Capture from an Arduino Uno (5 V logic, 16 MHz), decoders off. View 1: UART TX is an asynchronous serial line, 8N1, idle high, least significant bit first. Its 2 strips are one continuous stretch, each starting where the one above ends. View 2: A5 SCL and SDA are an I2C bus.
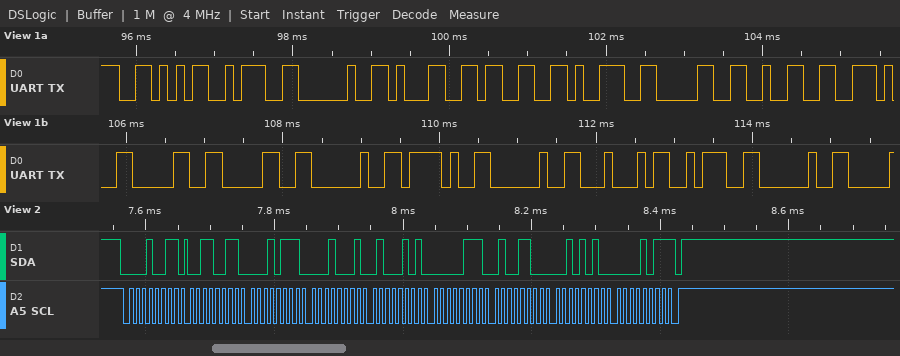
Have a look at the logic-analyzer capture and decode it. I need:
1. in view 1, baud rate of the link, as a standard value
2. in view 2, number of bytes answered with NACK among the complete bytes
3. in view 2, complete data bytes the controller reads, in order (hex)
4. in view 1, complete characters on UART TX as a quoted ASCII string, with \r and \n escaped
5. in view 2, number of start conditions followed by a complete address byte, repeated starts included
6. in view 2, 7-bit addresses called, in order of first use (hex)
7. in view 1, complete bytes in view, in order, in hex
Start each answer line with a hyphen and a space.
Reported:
- 9600 baud
- 1
- 33 17 11 45 07 4C 2A 0B
- "V: 13902.00 / D: "
- 1
- 0x09
- 56 3A 20 31 33 39 30 32 2E 30 30 20 2F 20 44 3A 20
